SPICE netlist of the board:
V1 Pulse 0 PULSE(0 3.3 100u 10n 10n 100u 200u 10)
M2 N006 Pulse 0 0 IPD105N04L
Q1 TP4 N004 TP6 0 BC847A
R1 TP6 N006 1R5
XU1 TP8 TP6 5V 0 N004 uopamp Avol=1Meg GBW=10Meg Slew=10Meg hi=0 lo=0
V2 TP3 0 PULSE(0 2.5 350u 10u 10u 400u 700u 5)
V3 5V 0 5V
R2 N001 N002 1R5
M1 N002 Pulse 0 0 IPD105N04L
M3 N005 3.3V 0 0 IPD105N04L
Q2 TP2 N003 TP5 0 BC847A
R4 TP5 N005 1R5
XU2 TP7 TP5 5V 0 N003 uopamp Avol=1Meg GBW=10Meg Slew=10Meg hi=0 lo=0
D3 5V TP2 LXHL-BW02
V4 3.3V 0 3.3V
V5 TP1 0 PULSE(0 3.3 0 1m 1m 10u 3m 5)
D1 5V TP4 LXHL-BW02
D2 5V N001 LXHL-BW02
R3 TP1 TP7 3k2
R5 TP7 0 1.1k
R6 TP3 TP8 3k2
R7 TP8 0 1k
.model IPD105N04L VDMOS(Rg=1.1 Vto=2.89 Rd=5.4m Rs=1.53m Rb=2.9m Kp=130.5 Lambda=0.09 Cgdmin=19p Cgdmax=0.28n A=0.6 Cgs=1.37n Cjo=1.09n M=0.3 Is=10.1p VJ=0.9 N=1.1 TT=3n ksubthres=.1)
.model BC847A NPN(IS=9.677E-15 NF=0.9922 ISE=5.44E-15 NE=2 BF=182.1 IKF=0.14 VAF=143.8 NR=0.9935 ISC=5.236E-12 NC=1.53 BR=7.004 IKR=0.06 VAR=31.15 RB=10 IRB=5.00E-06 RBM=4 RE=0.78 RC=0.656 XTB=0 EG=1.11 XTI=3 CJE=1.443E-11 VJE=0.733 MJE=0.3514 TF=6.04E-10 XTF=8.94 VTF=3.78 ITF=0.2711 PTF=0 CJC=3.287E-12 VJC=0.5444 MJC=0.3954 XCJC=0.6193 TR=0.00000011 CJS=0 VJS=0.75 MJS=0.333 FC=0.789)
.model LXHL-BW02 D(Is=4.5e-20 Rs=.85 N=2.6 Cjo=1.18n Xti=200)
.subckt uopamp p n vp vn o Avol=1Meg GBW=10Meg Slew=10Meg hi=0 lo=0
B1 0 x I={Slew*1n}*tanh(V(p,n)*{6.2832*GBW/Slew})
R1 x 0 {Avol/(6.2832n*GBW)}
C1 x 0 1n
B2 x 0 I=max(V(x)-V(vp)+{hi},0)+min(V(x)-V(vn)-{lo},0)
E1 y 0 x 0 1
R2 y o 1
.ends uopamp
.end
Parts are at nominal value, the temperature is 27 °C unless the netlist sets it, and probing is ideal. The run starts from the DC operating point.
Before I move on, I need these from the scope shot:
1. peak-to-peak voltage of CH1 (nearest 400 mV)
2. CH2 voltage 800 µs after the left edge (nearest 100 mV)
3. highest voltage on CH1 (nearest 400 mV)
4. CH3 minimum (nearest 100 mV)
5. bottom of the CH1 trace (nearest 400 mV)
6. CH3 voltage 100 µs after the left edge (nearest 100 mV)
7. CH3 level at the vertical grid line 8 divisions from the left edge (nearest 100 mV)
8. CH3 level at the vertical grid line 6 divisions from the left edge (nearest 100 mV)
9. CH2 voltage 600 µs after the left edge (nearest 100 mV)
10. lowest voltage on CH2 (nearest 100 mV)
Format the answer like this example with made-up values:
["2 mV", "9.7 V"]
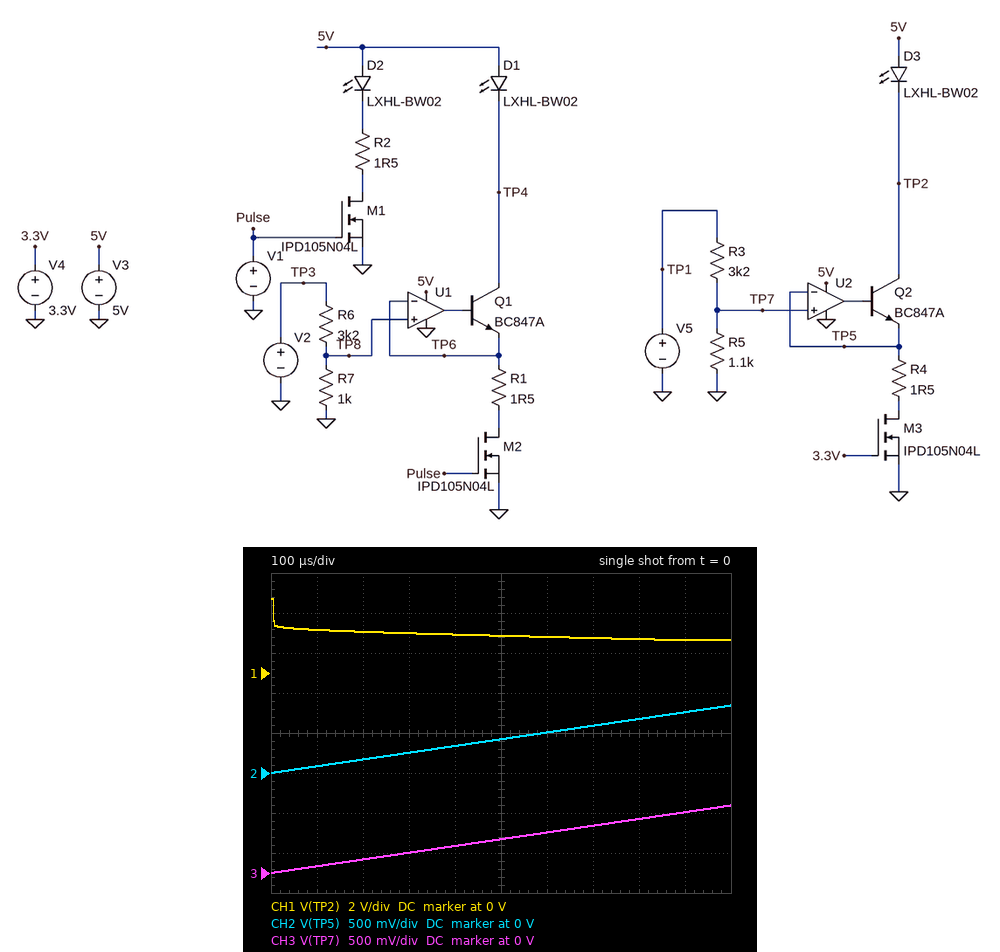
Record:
["2.0 V", "700 mV", "3.6 V", "0 V", "1.6 V", "100 mV", "700 mV", "500 mV", "500 mV", "0 V"]
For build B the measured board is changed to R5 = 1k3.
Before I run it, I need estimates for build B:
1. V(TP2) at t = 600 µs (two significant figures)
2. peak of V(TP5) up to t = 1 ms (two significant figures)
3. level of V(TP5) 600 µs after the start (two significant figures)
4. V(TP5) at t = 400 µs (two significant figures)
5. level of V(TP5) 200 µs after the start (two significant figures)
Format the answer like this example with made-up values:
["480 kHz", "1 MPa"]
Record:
["1.8 V", "950 mV", "570 mV", "380 mV", "190 mV"]
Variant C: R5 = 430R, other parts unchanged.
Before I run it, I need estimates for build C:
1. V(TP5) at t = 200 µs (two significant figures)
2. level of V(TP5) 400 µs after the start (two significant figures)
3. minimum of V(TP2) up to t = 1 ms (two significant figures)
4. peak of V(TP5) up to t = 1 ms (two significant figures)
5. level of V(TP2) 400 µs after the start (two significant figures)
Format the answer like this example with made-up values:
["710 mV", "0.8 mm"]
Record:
["78 mV", "160 mV", "1.9 V", "390 mV", "2.1 V"]
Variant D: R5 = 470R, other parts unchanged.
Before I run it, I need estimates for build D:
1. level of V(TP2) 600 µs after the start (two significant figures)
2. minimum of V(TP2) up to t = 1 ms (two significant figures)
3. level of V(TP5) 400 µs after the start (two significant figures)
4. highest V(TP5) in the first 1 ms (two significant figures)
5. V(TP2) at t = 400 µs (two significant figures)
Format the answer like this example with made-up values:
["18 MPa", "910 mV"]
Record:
["2.0 V", "1.9 V", "170 mV", "420 mV", "2.1 V"]
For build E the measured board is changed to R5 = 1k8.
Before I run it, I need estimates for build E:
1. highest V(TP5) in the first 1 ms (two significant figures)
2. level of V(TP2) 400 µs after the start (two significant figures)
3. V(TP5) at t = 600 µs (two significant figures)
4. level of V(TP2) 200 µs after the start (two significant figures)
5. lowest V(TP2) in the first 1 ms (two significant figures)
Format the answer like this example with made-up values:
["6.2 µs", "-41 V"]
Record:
["1.1 V", "1.8 V", "710 mV", "2.0 V", "1.6 V"]
